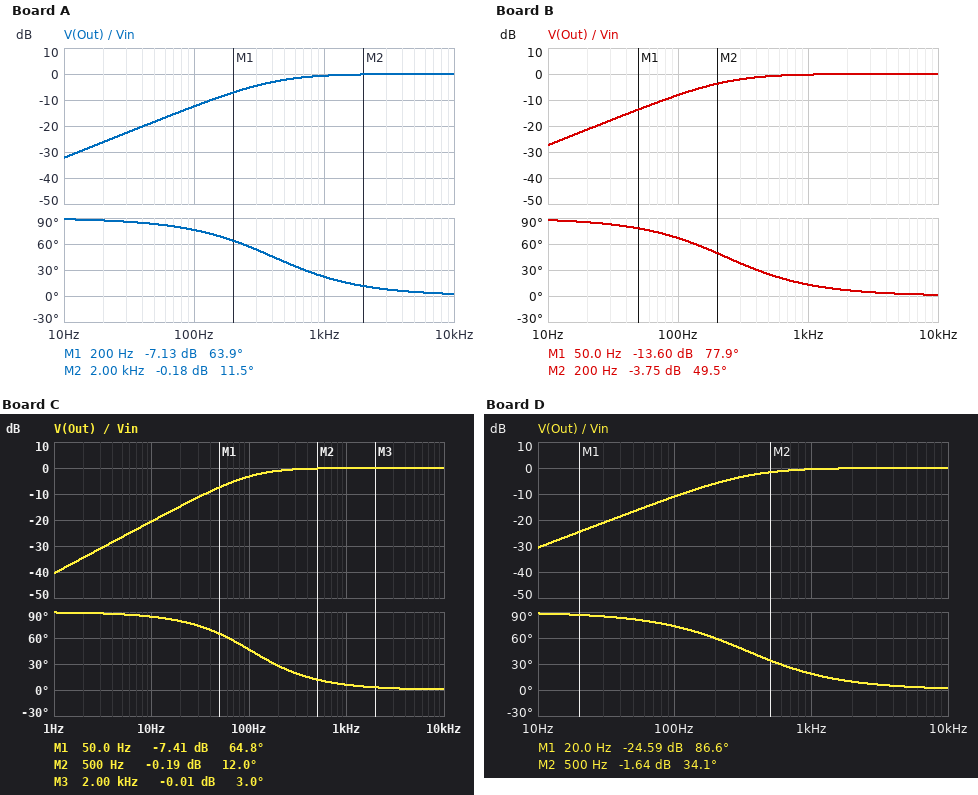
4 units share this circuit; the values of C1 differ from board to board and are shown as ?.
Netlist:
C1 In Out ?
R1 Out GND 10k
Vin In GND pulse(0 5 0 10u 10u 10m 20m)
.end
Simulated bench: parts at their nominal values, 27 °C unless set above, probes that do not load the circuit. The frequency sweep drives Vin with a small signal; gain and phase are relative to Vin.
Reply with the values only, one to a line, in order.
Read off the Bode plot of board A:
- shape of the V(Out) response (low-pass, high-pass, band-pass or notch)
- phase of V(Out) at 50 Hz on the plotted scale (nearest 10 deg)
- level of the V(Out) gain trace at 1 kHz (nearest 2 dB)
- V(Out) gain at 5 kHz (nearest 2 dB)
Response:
high-pass
80 deg
0 dB
0 dB
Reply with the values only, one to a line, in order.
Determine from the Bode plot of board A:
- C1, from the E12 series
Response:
39 nF
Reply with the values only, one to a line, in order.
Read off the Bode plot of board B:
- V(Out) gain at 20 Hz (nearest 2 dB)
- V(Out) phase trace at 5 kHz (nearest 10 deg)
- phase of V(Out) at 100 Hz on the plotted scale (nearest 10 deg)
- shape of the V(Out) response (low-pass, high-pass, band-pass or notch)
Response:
-22 dB
0 deg
70 deg
high-pass
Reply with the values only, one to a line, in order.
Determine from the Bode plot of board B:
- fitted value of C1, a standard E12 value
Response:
68 nF
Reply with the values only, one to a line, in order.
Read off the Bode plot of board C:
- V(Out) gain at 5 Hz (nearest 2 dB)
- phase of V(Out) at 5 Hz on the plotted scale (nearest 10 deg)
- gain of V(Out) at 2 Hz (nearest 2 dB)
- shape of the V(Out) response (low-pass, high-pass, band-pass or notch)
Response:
-26 dB
90 deg
-34 dB
high-pass
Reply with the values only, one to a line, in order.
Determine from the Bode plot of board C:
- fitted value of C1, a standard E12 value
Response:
150 nF
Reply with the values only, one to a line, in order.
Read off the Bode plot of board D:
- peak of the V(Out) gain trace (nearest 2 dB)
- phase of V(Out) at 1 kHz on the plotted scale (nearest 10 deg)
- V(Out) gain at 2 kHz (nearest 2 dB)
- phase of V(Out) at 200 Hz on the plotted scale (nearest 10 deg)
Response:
0 dB
20 deg
0 dB
60 deg
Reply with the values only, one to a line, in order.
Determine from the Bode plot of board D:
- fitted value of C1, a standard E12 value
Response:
47 nF
